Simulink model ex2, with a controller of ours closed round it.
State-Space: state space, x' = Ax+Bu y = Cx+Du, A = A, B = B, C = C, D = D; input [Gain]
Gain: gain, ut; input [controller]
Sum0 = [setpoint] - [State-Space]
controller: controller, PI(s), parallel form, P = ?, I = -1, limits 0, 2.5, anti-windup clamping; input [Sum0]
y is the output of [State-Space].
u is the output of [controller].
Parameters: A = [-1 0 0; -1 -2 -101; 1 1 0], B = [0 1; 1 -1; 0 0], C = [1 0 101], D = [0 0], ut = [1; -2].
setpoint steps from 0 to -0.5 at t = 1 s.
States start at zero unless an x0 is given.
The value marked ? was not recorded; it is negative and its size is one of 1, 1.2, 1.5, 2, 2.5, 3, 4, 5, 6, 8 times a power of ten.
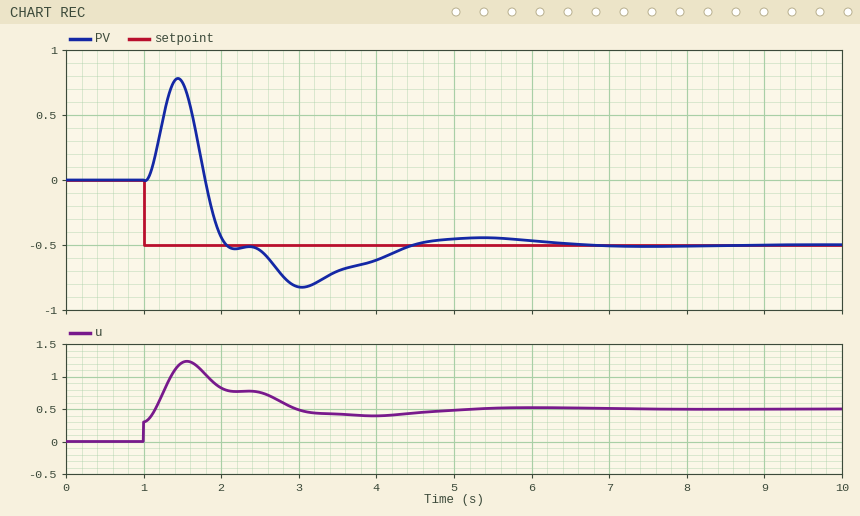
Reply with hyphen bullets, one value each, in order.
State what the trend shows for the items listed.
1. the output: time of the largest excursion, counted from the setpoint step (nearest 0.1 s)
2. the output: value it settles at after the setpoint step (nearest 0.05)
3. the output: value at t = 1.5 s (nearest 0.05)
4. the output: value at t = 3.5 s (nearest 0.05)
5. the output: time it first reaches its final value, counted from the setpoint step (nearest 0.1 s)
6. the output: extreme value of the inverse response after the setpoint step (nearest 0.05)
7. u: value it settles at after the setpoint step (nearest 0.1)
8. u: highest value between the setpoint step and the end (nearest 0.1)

- 2.0 s
- -0.50
- 0.75
- -0.70
- 1.1 s
- 0.80
- 0.5
- 1.2
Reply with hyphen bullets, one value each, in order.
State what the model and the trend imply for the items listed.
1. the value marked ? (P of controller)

- -0.6
